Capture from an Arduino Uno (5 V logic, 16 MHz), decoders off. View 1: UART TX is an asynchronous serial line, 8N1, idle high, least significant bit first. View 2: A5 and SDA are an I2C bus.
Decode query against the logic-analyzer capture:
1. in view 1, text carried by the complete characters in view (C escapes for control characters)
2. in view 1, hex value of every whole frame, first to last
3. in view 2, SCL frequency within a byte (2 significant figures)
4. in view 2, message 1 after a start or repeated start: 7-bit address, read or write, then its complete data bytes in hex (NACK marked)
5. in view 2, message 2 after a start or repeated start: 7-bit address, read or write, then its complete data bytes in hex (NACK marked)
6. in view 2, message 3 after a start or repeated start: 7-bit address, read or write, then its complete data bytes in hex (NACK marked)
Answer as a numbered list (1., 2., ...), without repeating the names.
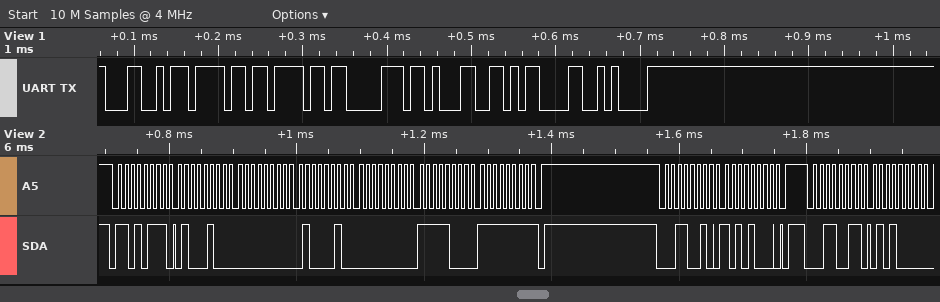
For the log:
1. "Loop1\r\n"
2. 4C 6F 6F 70 31 0D 0A
3. 100 kHz
4. 0x6B read: 44 00 42 00 F8 FF NACK
5. 0x19 write: A8
6. 0x19 read: 50
